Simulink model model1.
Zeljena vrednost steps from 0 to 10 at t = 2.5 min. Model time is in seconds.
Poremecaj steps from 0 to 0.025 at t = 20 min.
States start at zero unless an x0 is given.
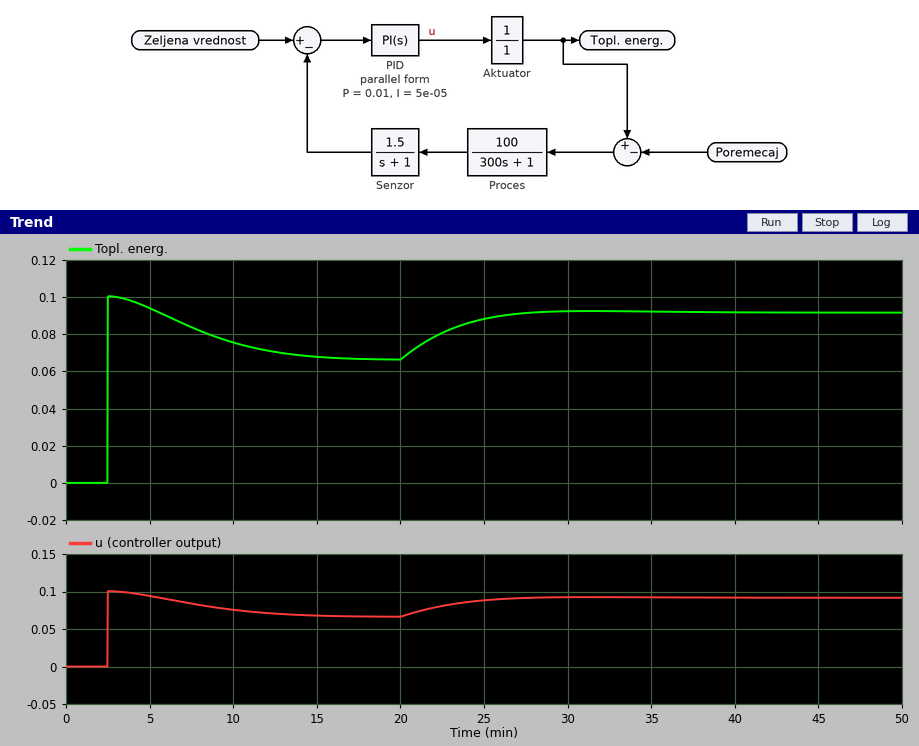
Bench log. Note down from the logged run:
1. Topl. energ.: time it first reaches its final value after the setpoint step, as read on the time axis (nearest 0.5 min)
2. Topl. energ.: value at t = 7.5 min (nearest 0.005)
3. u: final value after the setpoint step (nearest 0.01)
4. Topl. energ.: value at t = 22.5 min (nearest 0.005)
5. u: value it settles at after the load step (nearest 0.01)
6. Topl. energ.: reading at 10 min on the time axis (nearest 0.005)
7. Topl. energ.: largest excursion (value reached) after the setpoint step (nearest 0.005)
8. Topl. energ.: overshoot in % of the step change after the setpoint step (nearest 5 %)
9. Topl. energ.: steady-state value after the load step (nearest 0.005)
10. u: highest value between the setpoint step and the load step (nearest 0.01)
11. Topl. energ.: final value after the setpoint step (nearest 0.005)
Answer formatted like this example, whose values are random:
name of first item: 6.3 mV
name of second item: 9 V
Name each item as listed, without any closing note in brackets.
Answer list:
Topl. energ.: time it first reaches its final value after the setpoint step, as read on the time axis: 2.5 min
Topl. energ.: value at t = 7.5 min: 0.085
u: final value after the setpoint step: 0.07
Topl. energ.: value at t = 22.5 min: 0.080
u: value it settles at after the load step: 0.09
Topl. energ.: reading at 10 min on the time axis: 0.075
Topl. energ.: largest excursion (value reached) after the setpoint step: 0.100
Topl. energ.: overshoot in % of the step change after the setpoint step: 50 %
Topl. energ.: steady-state value after the load step: 0.090
u: highest value between the setpoint step and the load step: 0.10
Topl. energ.: final value after the setpoint step: 0.065
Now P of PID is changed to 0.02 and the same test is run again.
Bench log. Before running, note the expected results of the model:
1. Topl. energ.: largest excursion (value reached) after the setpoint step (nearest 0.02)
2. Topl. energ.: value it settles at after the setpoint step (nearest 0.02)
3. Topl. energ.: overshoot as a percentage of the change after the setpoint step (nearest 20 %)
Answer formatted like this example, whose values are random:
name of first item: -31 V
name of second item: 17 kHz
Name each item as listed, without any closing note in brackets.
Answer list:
Topl. energ.: largest excursion (value reached) after the setpoint step: 0.20
Topl. energ.: value it settles at after the setpoint step: 0.06
Topl. energ.: overshoot as a percentage of the change after the setpoint step: 200 %
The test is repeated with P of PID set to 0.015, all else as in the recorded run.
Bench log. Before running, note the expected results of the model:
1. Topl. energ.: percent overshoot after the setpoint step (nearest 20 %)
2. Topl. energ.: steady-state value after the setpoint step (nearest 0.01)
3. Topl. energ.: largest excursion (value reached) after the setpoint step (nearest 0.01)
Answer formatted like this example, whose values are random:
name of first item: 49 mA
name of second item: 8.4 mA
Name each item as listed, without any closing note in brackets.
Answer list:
Topl. energ.: percent overshoot after the setpoint step: 120 %
Topl. energ.: steady-state value after the setpoint step: 0.07
Topl. energ.: largest excursion (value reached) after the setpoint step: 0.15
